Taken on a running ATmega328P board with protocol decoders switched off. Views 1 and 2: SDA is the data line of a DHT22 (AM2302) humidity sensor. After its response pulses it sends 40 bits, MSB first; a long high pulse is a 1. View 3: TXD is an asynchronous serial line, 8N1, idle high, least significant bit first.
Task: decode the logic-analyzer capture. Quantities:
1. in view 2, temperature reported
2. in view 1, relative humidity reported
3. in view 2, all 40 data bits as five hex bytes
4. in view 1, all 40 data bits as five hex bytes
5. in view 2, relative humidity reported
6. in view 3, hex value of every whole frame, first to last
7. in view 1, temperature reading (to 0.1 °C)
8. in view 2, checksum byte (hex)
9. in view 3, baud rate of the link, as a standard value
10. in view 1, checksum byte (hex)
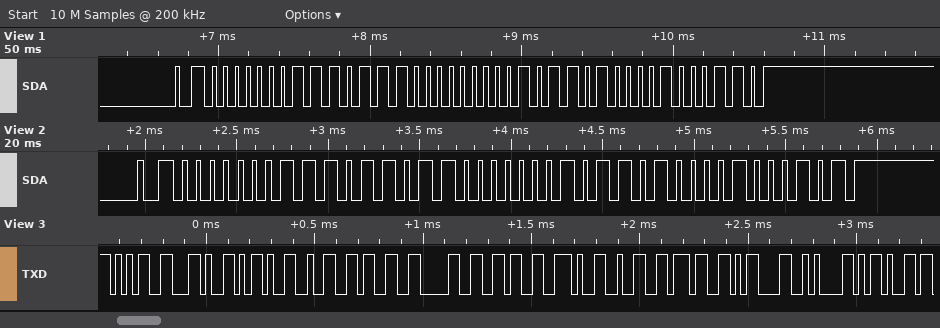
36.0 °C
47.6 %
01 DB 01 68 45
01 DC 01 68 46
47.5 %
0x35 0x2C 0x2D 0x32 0x33 0x30 0x36 0x2E 0x32 0x37 0x0D 0x0A 0x2D
36.0 °C
0x45
38400 baud
0x46
